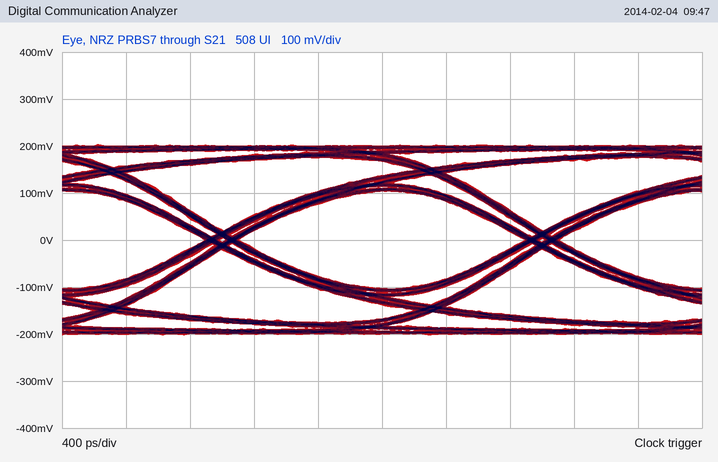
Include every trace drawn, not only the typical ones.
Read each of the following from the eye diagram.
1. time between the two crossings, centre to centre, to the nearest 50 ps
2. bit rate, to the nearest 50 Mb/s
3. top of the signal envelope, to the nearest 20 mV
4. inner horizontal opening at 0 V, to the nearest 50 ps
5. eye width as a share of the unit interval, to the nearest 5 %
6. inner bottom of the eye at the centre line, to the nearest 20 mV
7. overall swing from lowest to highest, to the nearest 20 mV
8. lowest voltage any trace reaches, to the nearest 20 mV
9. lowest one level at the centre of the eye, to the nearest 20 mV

2.00 ns
500 Mb/s
200 mV
1.80 ns
90 %
-100 mV
400 mV
-200 mV
100 mV
